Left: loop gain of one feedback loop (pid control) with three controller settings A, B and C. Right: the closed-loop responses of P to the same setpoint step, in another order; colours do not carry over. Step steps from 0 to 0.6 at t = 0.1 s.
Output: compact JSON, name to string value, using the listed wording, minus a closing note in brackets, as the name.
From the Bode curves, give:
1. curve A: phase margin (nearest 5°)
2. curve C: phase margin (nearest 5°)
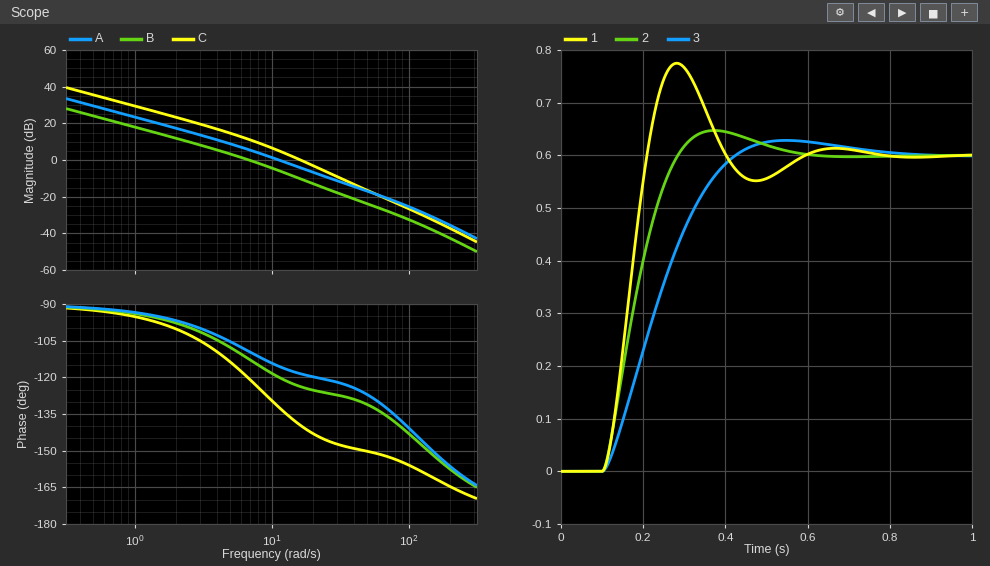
{"curve A: phase margin": "65°", "curve C: phase margin": "40°"}
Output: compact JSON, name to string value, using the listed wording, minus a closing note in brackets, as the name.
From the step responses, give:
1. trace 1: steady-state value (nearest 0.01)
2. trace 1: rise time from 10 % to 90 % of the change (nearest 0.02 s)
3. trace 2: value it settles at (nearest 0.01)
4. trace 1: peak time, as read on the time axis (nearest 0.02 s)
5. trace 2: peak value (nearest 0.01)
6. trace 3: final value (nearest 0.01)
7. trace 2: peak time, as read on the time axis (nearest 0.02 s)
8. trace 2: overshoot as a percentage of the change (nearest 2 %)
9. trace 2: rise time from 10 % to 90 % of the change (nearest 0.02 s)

{"trace 1: steady-state value": "0.60", "trace 1: rise time from 10 % to 90 % of the change": "0.08 s", "trace 2: value it settles at": "0.60", "trace 1: peak time, as read on the time axis": "0.28 s", "trace 2: peak value": "0.65", "trace 3: final value": "0.60", "trace 2: peak time, as read on the time axis": "0.38 s", "trace 2: overshoot as a percentage of the change": "8 %", "trace 2: rise time from 10 % to 90 % of the change": "0.12 s"}
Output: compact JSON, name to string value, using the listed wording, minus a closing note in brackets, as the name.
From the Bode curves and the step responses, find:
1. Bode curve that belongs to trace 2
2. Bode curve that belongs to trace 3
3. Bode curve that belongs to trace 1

{"Bode curve that belongs to trace 2": "A", "Bode curve that belongs to trace 3": "B", "Bode curve that belongs to trace 1": "C"}
